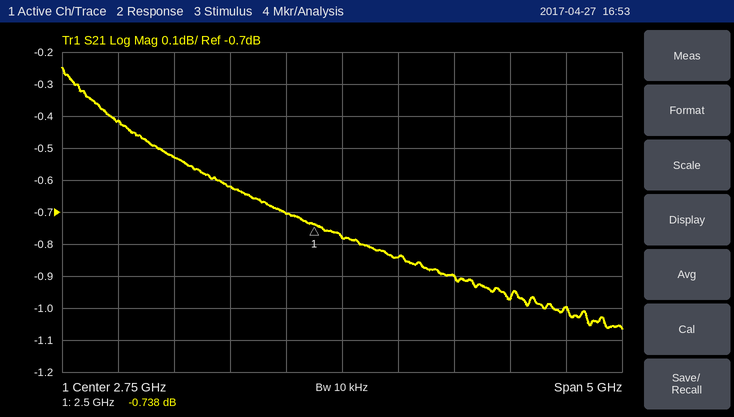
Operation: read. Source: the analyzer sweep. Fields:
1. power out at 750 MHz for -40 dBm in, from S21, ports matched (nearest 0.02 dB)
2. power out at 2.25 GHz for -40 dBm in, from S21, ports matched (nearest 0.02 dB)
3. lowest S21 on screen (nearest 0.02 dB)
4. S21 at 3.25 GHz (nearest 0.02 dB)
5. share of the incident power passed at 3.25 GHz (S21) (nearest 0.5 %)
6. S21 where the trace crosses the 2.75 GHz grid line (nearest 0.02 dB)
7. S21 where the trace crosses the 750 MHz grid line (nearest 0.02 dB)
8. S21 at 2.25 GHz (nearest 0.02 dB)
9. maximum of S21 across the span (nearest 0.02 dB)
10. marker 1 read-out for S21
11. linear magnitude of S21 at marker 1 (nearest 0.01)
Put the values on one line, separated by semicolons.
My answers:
-40.42 dBm; -40.70 dBm; -1.06 dB; -0.84 dB; 82.5 %; -0.78 dB; -0.42 dB; -0.70 dB; -0.24 dB; -0.738 dB; 0.92
